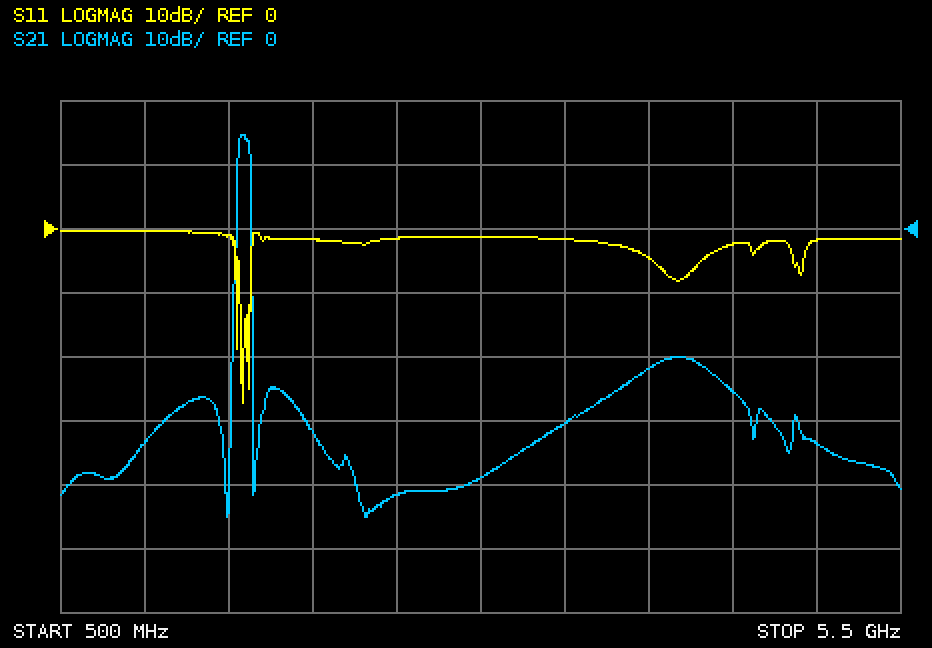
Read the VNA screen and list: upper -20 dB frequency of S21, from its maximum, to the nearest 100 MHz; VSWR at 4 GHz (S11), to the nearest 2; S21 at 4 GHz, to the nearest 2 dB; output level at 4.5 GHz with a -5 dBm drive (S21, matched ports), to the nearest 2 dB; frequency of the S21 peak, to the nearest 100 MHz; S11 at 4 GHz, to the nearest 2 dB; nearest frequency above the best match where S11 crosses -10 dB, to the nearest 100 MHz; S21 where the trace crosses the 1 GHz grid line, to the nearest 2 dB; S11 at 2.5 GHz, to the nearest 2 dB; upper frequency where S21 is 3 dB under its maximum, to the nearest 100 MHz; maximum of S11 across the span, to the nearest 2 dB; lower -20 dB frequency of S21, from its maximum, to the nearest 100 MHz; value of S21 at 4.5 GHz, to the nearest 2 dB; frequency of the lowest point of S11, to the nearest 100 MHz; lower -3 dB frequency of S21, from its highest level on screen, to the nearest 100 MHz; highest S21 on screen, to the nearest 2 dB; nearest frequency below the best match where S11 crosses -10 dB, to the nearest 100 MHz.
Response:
1.6 GHz
4
-22 dB
-30 dBm
1.6 GHz
-4 dB
1.6 GHz
-34 dB
-2 dB
1.6 GHz
0 dB
1.5 GHz
-26 dB
1.6 GHz
1.6 GHz
14 dB
1.6 GHz
